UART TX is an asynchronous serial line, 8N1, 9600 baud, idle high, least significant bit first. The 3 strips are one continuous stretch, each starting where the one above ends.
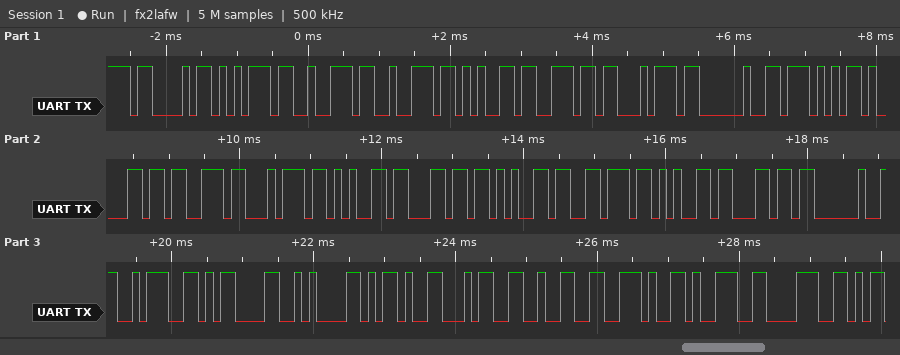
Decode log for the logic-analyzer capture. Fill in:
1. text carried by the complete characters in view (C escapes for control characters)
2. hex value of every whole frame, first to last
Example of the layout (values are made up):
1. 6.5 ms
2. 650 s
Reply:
1. "Current Wastelevel :\r\n-42.98"
2. 43 75 72 72 65 6E 74 20 57 61 73 74 65 6C 65 76 65 6C 20 3A 0D 0A 2D 34 32 2E 39 38
